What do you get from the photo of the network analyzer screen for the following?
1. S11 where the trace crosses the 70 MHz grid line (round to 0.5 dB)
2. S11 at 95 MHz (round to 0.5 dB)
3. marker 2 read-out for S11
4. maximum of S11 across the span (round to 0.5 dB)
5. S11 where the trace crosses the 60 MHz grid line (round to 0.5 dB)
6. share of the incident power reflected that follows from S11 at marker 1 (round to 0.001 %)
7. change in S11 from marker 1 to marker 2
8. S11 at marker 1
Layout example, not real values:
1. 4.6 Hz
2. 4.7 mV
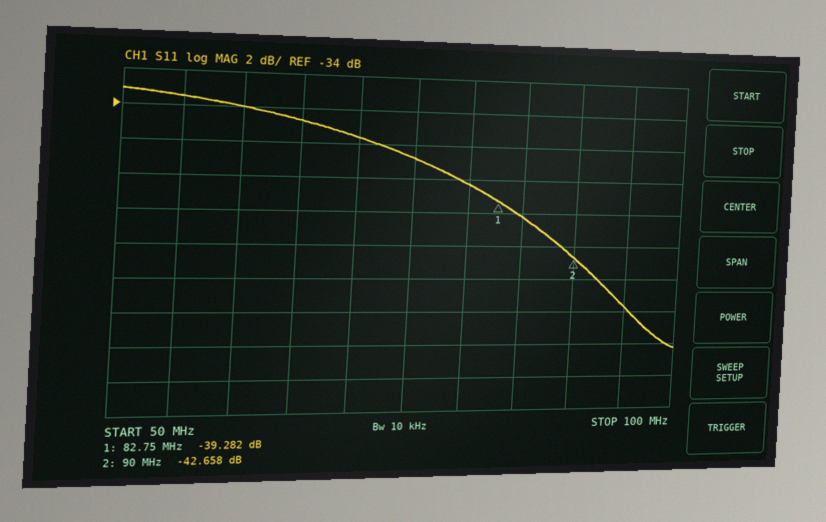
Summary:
1. -35.5 dB
2. -45.5 dB
3. -42.658 dB
4. -33.0 dB
5. -34.0 dB
6. 0.012 %
7. -3.376 dB
8. -39.282 dB
